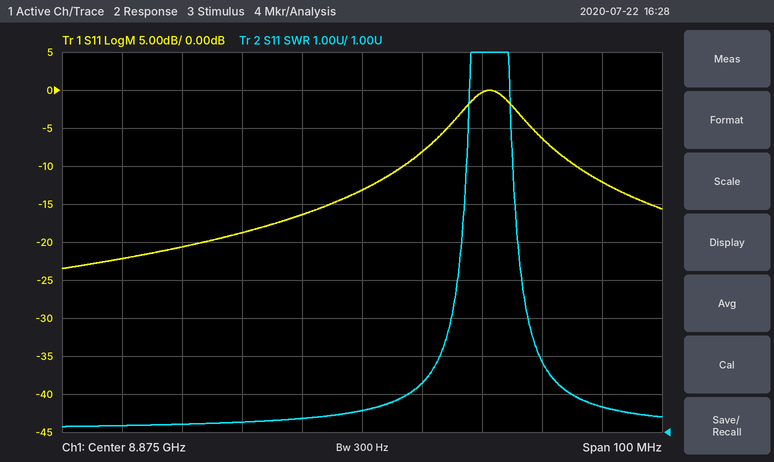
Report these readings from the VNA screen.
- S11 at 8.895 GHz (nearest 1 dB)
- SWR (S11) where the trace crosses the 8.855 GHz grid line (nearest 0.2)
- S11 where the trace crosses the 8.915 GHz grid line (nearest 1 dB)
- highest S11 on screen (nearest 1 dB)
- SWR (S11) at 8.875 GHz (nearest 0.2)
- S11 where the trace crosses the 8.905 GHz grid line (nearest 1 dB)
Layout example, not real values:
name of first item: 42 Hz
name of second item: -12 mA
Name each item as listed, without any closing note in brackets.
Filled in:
S11 at 8.895 GHz: 0 dB
SWR (S11) where the trace crosses the 8.855 GHz grid line: 1.2
S11 where the trace crosses the 8.915 GHz grid line: -12 dB
highest S11 on screen: 0 dB
SWR (S11) at 8.875 GHz: 1.6
S11 where the trace crosses the 8.905 GHz grid line: -6 dB
